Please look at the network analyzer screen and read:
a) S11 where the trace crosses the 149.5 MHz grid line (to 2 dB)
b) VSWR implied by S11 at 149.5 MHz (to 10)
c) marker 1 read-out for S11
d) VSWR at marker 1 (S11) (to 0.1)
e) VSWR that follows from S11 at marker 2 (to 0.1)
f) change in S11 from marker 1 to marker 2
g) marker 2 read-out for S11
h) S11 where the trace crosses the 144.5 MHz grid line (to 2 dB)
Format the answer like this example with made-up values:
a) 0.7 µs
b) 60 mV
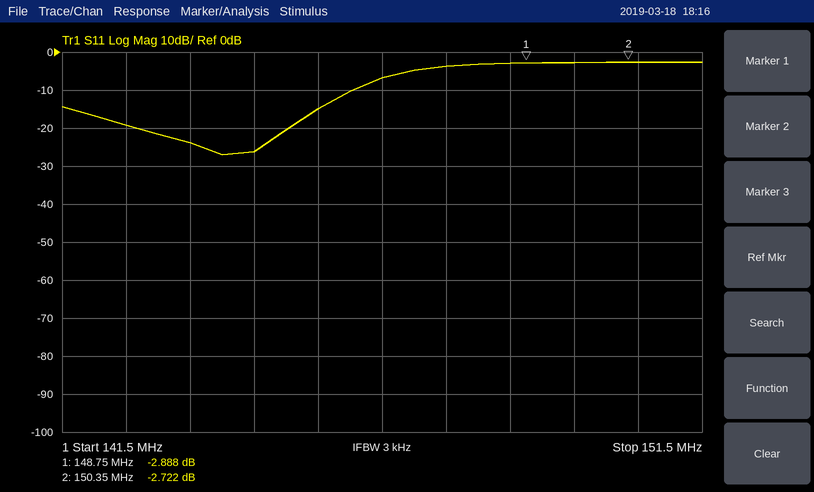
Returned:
a) -2 dB
b) 10
c) -2.888 dB
d) 6.1
e) 6.4
f) 0.166 dB
g) -2.722 dB
h) -26 dB
